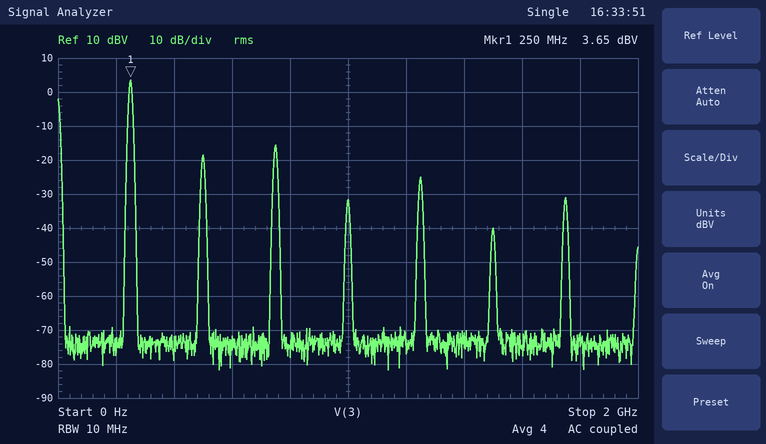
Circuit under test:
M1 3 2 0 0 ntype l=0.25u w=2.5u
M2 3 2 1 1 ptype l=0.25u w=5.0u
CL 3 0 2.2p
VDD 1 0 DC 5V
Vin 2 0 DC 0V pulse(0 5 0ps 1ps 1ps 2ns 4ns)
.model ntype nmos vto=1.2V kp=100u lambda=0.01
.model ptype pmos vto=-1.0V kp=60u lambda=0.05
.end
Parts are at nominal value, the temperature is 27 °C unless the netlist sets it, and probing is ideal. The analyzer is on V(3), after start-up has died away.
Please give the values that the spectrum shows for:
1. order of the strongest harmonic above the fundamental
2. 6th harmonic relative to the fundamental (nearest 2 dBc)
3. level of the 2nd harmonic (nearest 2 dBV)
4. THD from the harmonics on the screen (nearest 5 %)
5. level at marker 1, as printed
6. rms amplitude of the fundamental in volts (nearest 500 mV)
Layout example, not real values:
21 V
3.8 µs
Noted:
3
-44 dBc
-18 dBV
15 %
3.65 dBV
1.5 V
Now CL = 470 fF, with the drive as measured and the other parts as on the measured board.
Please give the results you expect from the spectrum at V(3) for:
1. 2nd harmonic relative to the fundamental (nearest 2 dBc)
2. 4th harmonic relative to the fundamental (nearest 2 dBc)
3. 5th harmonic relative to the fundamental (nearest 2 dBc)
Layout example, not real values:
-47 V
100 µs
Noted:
-28 dBc
-30 dBc
-18 dBc
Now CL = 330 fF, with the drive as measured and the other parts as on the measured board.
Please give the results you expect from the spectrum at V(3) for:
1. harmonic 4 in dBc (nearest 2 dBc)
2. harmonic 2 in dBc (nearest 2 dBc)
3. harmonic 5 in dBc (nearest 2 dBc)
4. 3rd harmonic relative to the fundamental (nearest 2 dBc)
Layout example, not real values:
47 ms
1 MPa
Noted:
-32 dBc
-30 dBc
-16 dBc
-10 dBc
